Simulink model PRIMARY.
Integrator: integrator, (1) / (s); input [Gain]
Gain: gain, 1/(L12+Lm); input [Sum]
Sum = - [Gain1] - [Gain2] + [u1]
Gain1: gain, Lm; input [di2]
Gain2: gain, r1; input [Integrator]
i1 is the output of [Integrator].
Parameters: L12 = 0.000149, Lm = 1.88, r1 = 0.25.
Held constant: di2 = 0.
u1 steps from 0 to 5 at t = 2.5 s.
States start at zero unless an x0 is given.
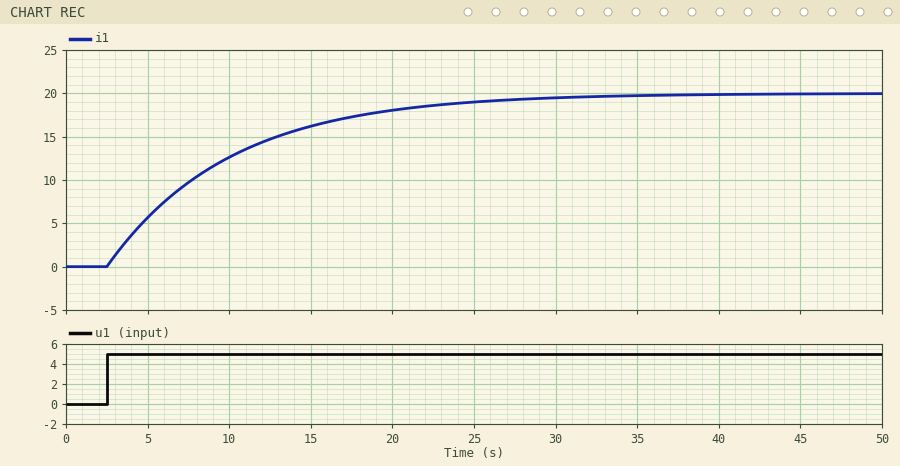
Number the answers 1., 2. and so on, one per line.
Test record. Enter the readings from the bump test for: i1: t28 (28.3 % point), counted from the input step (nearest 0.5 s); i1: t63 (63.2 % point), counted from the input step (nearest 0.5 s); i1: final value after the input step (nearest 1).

1. 2.5 s
2. 7.5 s
3. 20
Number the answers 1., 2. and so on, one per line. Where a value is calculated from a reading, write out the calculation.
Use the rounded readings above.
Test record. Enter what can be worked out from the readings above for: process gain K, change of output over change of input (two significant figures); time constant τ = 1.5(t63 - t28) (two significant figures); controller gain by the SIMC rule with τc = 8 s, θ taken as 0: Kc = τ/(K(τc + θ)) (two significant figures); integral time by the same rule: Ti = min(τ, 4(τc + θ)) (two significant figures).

1. (20 - 0) / 5 = 4.0
2. 1.5 × (7.5 - 2.5) = 7.5 s
3. 7.5 / (4 × (8 + 0)) = 0.23
4. min(7.5, 4 × (8 + 0)) = 7.5 s
